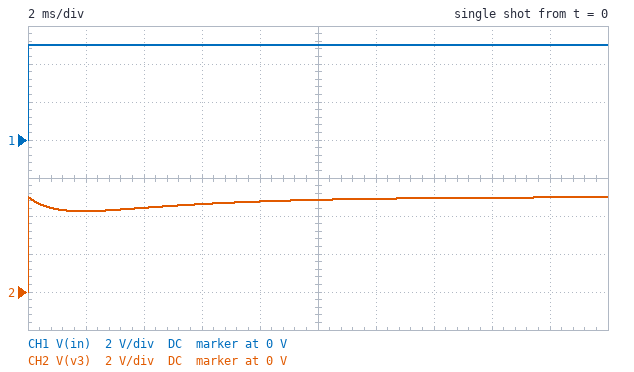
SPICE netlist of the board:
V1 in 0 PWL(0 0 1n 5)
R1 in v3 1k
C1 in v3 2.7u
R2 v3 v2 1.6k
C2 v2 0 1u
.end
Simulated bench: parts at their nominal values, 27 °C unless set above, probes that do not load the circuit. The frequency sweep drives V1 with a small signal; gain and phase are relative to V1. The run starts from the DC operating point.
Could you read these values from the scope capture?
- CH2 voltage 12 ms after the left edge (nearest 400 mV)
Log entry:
4.8 V
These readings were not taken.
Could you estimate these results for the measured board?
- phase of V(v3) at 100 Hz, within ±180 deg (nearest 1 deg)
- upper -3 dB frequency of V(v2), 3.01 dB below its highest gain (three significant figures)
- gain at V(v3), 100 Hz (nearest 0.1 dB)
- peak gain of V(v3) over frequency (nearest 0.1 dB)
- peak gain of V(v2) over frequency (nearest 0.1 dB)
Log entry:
3 deg
58.5 Hz
-1.7 dB
0 dB
0 dB
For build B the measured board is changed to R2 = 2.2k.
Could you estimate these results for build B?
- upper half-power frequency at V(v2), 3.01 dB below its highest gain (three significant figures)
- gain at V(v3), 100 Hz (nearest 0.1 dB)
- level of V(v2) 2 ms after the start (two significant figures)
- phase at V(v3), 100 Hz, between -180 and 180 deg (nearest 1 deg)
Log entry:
47.1 Hz
-1.4 dB
2.7 V
4 deg
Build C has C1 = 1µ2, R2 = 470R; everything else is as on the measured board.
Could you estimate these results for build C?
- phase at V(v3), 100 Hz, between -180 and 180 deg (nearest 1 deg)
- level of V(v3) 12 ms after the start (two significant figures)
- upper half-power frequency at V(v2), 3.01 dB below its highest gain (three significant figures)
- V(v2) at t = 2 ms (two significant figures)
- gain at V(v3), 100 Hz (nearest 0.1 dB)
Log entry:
-12 deg
5.0 V
88.7 Hz
3.8 V
-3.0 dB
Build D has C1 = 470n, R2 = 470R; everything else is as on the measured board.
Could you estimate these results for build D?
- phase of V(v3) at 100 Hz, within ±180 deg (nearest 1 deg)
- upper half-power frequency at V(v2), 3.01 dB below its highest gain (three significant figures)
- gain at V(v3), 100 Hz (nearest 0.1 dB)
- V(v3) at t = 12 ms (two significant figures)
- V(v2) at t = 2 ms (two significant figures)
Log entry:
-20 deg
93.5 Hz
-2.9 dB
5.0 V
3.7 V
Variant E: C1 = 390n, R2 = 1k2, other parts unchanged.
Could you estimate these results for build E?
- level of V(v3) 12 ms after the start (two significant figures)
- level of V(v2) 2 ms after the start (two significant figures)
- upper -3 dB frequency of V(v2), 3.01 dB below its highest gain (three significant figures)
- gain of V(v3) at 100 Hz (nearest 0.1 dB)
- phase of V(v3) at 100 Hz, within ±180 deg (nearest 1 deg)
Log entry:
5.0 V
3.0 V
67.8 Hz
-3.0 dB
-13 deg
